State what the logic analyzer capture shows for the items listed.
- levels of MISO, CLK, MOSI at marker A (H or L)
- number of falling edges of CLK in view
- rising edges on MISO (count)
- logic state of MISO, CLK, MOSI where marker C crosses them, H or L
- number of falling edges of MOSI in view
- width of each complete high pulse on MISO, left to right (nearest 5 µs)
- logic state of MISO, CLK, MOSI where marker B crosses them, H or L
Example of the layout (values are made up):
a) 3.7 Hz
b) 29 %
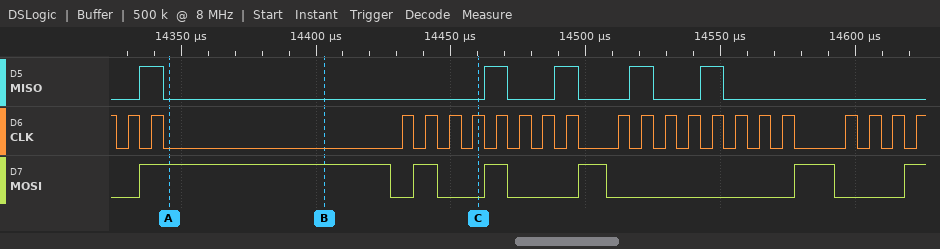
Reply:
a) MISO=L, CLK=L, MOSI=H
b) 22
c) 5
d) MISO=L, CLK=H, MOSI=L
e) 5
f) 10 µs, 10 µs, 10 µs, 10 µs, 10 µs
g) MISO=L, CLK=L, MOSI=H
